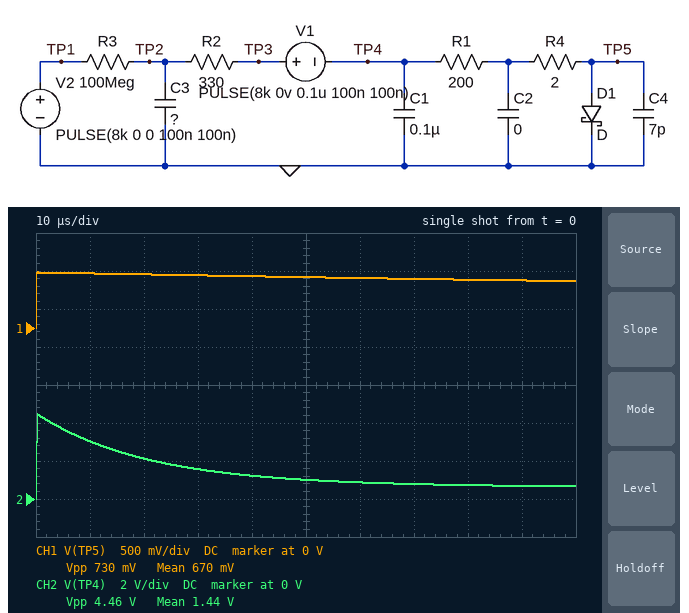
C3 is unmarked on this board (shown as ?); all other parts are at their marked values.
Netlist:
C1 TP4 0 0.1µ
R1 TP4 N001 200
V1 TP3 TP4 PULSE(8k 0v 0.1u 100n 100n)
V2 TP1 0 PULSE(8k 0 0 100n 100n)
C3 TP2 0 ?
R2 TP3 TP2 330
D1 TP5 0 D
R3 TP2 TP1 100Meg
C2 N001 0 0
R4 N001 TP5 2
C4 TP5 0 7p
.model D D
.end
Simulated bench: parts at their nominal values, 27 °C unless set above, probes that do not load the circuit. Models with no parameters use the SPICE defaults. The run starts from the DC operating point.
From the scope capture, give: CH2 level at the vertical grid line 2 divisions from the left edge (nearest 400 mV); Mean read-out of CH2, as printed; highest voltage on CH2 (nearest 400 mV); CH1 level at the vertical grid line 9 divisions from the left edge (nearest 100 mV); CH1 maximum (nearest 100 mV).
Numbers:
2.0 V
1.44 V
4.4 V
600 mV
700 mV
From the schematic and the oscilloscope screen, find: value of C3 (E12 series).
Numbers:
56 pF
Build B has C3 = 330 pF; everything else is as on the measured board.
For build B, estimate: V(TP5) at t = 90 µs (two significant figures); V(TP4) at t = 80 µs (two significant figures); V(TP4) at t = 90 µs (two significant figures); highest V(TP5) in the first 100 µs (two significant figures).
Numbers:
670 mV
1.2 V
1.0 V
780 mV
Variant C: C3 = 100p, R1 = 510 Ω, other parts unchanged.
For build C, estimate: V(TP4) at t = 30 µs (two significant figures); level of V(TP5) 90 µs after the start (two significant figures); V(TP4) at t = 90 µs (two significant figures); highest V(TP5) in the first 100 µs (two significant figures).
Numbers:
4.8 V
680 mV
2.0 V
720 mV
